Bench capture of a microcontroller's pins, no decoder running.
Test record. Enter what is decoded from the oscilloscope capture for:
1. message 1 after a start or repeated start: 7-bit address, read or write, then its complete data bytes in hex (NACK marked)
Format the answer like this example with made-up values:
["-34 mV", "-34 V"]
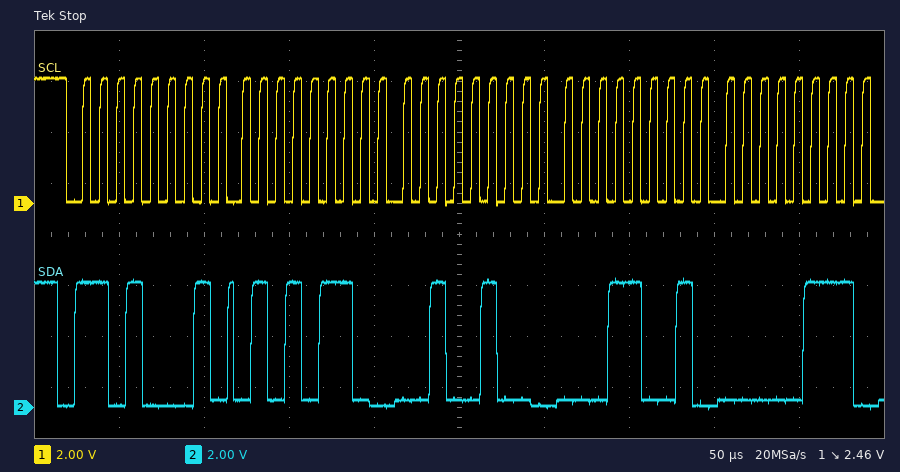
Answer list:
["0x68 read: 56 24 19 07"]
